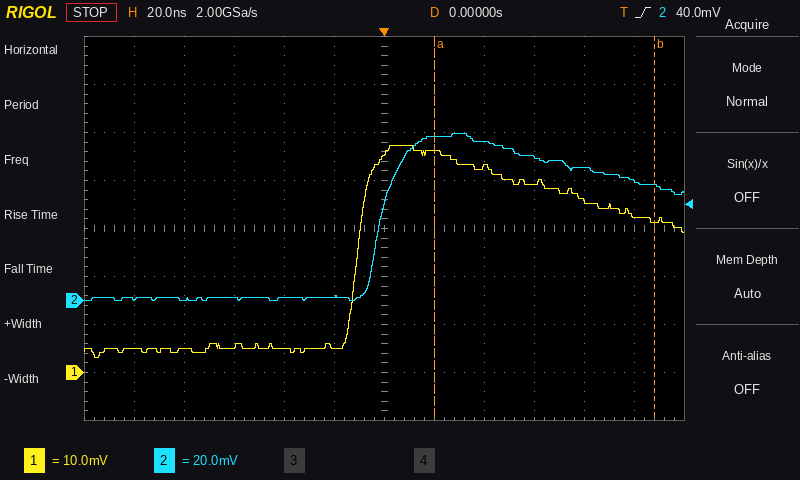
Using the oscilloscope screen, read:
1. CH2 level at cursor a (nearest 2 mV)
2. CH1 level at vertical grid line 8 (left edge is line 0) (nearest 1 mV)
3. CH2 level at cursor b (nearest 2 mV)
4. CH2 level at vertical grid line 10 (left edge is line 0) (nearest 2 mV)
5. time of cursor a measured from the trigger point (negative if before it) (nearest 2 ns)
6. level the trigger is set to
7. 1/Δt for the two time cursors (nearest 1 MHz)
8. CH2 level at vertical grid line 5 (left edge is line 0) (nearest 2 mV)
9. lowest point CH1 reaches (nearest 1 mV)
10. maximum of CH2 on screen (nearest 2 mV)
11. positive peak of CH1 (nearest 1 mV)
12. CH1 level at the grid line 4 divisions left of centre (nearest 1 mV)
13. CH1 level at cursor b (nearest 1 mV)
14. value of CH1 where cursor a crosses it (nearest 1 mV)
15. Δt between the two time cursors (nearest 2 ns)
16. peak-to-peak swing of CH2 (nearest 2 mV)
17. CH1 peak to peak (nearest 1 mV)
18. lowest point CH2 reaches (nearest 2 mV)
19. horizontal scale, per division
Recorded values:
68 mV
43 mV
48 mV
56 mV
+20 ns
40.0 mV
11 MHz
2 mV
3 mV
70 mV
47 mV
5 mV
31 mV
46 mV
88 ns
70 mV
44 mV
0 mV
20 ns
